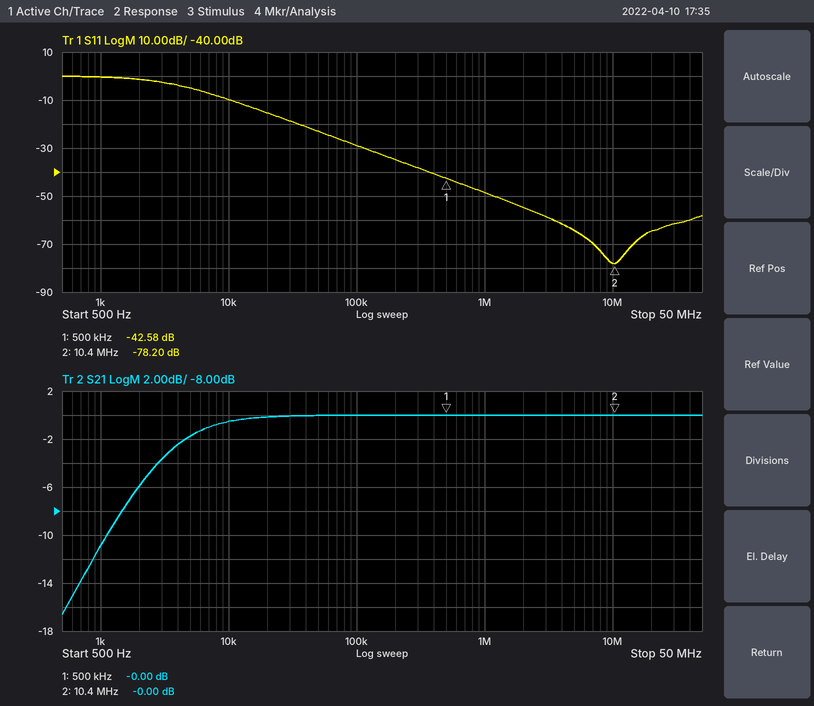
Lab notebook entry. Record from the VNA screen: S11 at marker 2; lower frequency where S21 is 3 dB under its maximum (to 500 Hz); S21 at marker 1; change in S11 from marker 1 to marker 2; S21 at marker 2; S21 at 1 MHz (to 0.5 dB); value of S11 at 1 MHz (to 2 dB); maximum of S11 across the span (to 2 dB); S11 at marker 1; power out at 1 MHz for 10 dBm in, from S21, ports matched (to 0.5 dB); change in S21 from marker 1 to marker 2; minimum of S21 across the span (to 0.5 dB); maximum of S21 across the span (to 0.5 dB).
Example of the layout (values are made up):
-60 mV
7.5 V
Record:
-78.20 dB
3.5 kHz
-0.00 dB
-35.62 dB
-0.00 dB
0.0 dB
-48 dB
0 dB
-42.58 dB
10.0 dBm
0.00 dB
-16.5 dB
0.0 dB
